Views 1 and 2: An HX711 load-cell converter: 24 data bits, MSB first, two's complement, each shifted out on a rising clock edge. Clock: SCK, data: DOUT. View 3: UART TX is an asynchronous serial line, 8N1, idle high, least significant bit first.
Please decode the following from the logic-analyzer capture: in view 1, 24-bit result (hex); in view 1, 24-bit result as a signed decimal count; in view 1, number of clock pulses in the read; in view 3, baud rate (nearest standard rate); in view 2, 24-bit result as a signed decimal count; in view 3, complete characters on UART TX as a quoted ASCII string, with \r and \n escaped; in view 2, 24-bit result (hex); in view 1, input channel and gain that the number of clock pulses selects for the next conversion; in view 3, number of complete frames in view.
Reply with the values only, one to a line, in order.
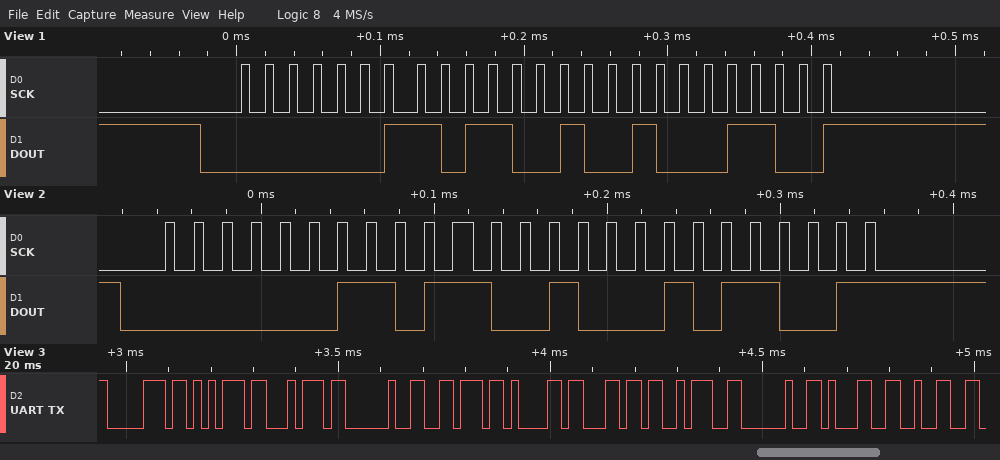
0x03648C
222348
25
57600 baud
222297
"put val: 12"
0x036459
channel A, gain 128
11
